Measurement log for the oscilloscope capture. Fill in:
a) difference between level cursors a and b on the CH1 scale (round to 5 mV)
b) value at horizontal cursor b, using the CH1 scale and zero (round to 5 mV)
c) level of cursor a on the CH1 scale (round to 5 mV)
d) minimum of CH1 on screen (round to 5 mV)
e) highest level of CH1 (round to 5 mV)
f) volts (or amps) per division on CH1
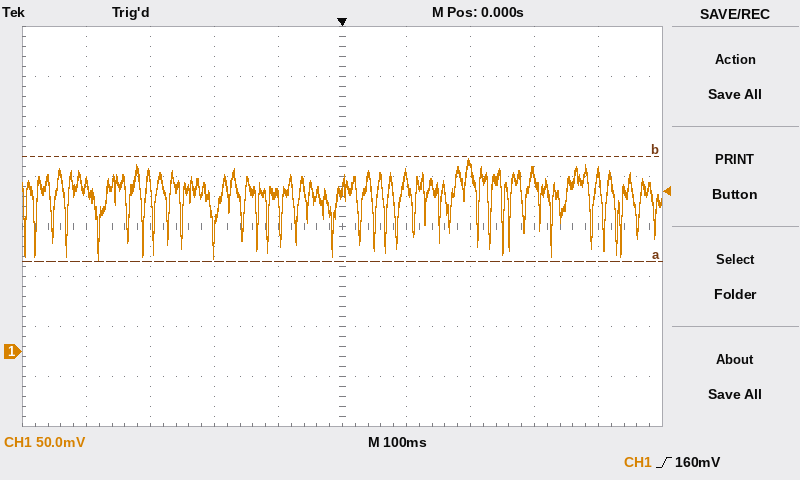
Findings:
105 mV
195 mV
90 mV
90 mV
195 mV
50 mV
